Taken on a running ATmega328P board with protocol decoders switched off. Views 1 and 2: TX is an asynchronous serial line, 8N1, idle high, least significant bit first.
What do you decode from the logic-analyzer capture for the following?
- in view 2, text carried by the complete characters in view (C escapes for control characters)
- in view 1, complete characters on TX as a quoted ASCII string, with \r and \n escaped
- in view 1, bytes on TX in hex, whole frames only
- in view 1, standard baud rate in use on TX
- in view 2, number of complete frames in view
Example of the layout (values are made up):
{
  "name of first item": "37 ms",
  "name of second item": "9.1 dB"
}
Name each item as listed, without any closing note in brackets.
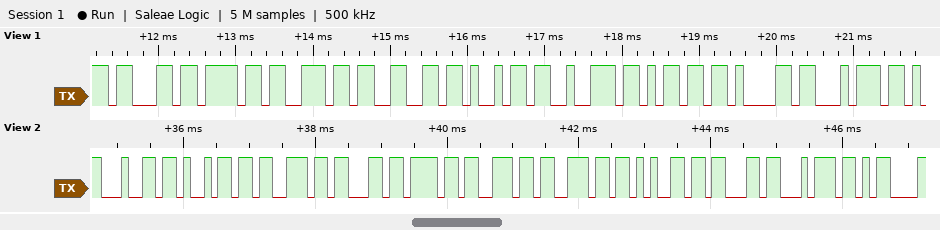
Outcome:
{
  "in view 2, text carried by the complete characters in view": "\"disconnect\\r\"",
  "in view 1, complete characters on TX as a quoted ASCII string, with \\r and \\n escaped": "\"confirmat\"",
  "in view 1, bytes on TX in hex, whole frames only": "0x63 0x6F 0x6E 0x66 0x69 0x72 0x6D 0x61 0x74",
  "in view 1, standard baud rate in use on TX": "9600 baud",
  "in view 2, number of complete frames in view": "11"
}
